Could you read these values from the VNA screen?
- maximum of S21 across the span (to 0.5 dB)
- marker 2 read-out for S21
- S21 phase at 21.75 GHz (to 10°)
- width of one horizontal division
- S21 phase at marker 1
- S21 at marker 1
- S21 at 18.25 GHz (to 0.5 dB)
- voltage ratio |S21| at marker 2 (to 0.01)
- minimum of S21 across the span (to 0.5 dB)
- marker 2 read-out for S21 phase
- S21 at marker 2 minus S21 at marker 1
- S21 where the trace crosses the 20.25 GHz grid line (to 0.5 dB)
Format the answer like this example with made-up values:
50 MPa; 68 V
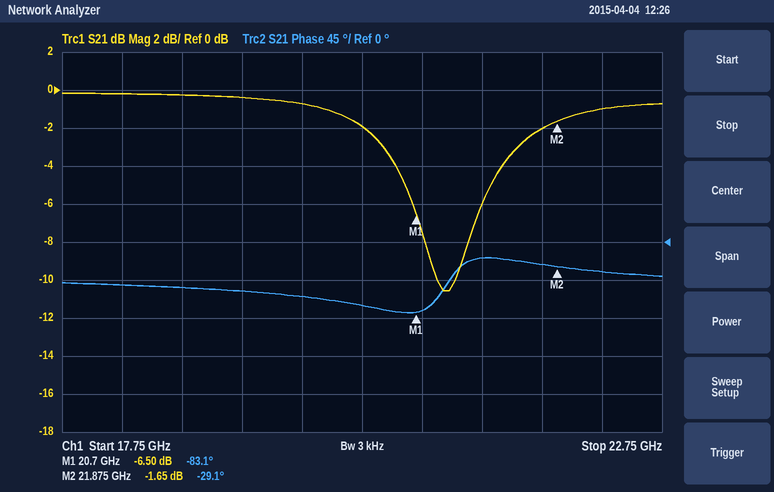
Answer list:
0.0 dB; -1.65 dB; -30°; 500 MHz; -83.1°; -6.50 dB; 0.0 dB; 0.83; -10.5 dB; -29.1°; 4.85 dB; -2.0 dB
